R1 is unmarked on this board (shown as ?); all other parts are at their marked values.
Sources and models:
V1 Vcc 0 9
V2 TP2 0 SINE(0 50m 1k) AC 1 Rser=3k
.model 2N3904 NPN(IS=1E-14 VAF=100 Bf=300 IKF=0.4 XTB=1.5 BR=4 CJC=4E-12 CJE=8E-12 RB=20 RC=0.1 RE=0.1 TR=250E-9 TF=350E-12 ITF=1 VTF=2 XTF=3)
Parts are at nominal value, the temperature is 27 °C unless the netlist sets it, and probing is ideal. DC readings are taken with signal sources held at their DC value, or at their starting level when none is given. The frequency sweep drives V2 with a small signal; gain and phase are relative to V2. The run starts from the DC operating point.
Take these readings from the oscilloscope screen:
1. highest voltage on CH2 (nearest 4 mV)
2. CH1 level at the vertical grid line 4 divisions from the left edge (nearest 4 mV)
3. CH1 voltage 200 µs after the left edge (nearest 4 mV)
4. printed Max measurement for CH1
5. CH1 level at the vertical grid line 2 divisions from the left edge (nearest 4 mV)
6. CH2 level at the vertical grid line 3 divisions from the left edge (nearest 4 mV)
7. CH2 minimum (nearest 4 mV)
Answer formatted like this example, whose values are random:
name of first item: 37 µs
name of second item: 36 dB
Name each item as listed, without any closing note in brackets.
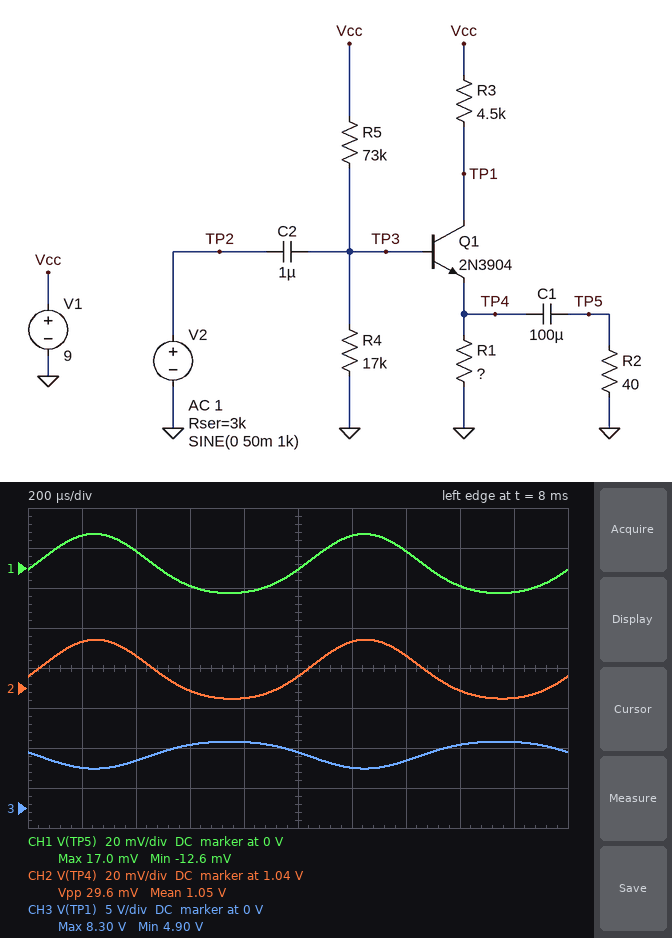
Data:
highest voltage on CH2: 1.064 V
CH1 level at the vertical grid line 4 divisions from the left edge: -12 mV
CH1 voltage 200 µs after the left edge: 16 mV
printed Max measurement for CH1: 17.0 mV
CH1 level at the vertical grid line 2 divisions from the left edge: 8 mV
CH2 level at the vertical grid line 3 divisions from the left edge: 1.040 V
CH2 minimum: 1.036 V
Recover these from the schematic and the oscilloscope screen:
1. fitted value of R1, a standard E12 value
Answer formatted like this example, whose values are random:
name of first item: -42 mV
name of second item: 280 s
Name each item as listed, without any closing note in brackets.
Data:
fitted value of R1, a standard E12 value: 2.2 kΩ
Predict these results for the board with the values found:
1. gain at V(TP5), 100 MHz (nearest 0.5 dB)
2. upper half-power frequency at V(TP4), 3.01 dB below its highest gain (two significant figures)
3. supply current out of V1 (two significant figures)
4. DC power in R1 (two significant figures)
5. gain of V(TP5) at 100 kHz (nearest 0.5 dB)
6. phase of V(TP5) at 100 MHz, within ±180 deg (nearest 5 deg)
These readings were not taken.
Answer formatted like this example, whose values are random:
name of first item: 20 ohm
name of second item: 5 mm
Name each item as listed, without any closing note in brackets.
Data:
gain at V(TP5), 100 MHz: -38.5 dB
upper half-power frequency at V(TP4), 3.01 dB below its highest gain: 110 Hz
supply current out of V1: 570 µA
DC power in R1: 500 µW
gain of V(TP5) at 100 kHz: -10.0 dB
phase of V(TP5) at 100 MHz, within ±180 deg: -5 deg
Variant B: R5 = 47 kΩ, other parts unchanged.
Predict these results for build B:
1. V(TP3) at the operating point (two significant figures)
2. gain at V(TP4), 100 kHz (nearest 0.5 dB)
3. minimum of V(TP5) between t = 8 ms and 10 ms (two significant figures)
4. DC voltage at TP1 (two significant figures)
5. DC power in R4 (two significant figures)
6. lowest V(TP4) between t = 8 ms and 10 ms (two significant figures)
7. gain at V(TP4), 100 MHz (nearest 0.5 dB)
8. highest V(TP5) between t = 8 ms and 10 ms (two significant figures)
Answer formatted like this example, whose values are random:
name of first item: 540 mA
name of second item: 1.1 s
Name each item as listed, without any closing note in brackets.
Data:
V(TP3) at the operating point: 2.4 V
gain at V(TP4), 100 kHz: -8.5 dB
minimum of V(TP5) between t = 8 ms and 10 ms: -17 mV
DC voltage at TP1: 5.5 V
DC power in R4: 330 µW
lowest V(TP4) between t = 8 ms and 10 ms: 1.7 V
gain at V(TP4), 100 MHz: -38.5 dB
highest V(TP5) between t = 8 ms and 10 ms: 20 mV
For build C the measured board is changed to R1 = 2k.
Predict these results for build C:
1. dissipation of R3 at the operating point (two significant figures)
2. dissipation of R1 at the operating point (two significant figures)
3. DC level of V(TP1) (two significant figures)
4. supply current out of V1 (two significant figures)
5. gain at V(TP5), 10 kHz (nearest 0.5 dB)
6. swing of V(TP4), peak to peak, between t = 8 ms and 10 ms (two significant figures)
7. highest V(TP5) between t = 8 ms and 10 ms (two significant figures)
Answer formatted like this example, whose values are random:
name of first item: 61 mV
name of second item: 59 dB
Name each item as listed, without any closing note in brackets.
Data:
dissipation of R3 at the operating point: 1.2 mW
dissipation of R1 at the operating point: 540 µW
DC level of V(TP1): 6.7 V
supply current out of V1: 620 µA
gain at V(TP5), 10 kHz: -9.5 dB
swing of V(TP4), peak to peak, between t = 8 ms and 10 ms: 31 mV
highest V(TP5) between t = 8 ms and 10 ms: 18 mV
